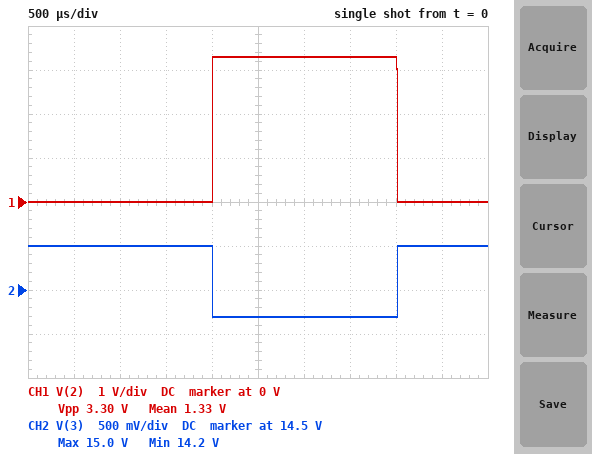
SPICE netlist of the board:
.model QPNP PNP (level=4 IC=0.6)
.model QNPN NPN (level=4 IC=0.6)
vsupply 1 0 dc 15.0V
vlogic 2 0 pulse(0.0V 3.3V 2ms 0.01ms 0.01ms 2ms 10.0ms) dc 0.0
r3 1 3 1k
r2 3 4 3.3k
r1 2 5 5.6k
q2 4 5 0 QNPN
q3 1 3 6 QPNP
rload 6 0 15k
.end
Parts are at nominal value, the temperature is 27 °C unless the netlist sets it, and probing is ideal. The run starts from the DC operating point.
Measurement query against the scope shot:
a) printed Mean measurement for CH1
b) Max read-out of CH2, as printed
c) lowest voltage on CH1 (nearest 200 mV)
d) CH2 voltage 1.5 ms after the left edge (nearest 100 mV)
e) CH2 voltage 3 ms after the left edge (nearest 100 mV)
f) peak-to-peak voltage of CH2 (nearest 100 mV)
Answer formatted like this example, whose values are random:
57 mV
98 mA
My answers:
1.33 V
15.0 V
0 V
15.0 V
14.2 V
800 mV
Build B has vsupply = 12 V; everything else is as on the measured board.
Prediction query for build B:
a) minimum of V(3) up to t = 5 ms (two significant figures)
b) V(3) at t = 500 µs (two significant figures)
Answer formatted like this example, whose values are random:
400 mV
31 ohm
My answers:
11 V
12 V
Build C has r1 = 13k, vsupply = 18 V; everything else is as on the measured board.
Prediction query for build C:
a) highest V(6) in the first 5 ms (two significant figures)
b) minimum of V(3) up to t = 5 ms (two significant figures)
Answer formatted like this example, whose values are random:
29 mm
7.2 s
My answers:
18 V
17 V
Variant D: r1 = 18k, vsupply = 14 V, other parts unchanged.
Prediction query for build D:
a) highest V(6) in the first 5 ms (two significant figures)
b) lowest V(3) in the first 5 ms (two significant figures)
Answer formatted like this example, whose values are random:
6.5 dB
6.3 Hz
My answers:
14 V
13 V
